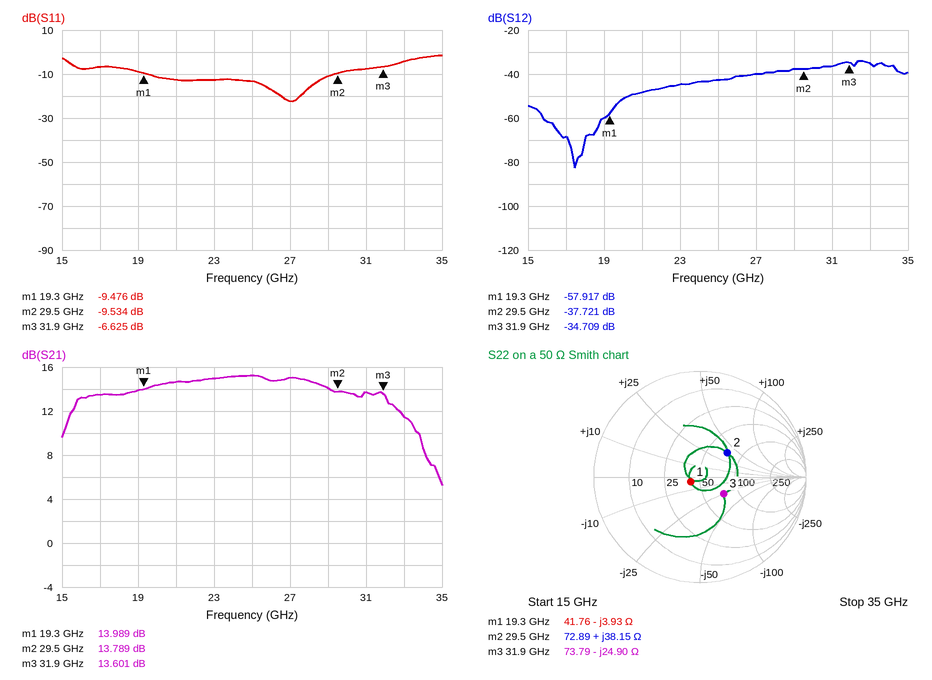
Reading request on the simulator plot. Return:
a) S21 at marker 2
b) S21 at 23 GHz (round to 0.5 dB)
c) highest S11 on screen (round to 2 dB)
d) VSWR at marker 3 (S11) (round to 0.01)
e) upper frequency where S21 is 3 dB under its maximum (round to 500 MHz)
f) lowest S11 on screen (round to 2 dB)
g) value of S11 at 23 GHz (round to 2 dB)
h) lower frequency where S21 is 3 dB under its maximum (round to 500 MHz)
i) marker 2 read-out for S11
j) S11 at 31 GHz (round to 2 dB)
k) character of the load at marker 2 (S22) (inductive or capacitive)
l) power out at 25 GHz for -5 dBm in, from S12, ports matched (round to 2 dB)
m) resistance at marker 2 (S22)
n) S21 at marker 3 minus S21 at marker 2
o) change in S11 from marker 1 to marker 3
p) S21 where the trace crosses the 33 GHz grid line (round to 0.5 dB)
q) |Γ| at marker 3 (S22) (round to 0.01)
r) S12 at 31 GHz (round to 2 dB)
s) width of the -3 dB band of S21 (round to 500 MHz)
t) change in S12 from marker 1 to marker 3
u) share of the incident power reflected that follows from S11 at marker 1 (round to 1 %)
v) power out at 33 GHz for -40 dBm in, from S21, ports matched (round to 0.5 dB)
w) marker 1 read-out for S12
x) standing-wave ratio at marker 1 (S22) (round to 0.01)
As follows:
13.789 dB
15.0 dB
-2 dB
2.75
32.5 GHz
-22 dB
-12 dB
15.5 GHz
-9.534 dB
-8 dB
inductive
-48 dBm
72.89 Ω
-0.188 dB
2.851 dB
11.5 dB
0.27
-36 dB
17.0 GHz
23.208 dB
11 %
-28.5 dBm
-57.917 dB
1.22
